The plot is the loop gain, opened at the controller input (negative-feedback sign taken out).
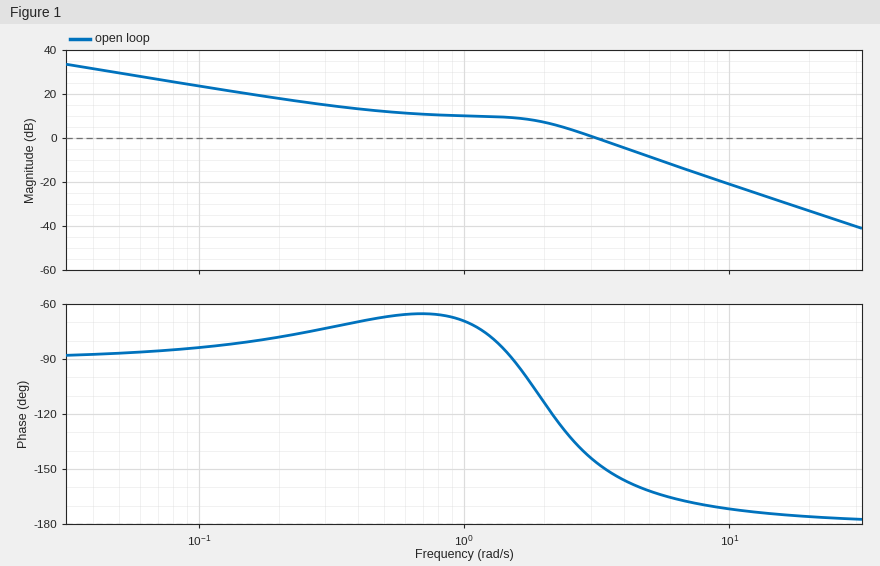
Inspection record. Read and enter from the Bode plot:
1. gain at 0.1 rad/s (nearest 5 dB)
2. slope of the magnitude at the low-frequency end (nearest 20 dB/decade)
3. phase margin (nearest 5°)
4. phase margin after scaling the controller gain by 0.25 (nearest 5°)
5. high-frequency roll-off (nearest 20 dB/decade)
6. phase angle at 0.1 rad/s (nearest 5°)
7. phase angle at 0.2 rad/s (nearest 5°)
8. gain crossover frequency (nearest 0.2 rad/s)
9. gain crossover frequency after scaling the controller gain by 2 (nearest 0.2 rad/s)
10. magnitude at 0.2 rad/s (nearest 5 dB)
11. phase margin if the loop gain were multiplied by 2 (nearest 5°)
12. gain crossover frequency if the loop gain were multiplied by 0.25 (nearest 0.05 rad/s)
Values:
25 dB
-20 dB/decade
35°
115°
-40 dB/decade
-85°
-80°
3.2 rad/s
4.4 rad/s
20 dB
20°
0.50 rad/s
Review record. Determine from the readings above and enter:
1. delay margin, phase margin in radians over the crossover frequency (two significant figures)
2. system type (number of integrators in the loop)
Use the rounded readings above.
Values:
0.19 s
1
